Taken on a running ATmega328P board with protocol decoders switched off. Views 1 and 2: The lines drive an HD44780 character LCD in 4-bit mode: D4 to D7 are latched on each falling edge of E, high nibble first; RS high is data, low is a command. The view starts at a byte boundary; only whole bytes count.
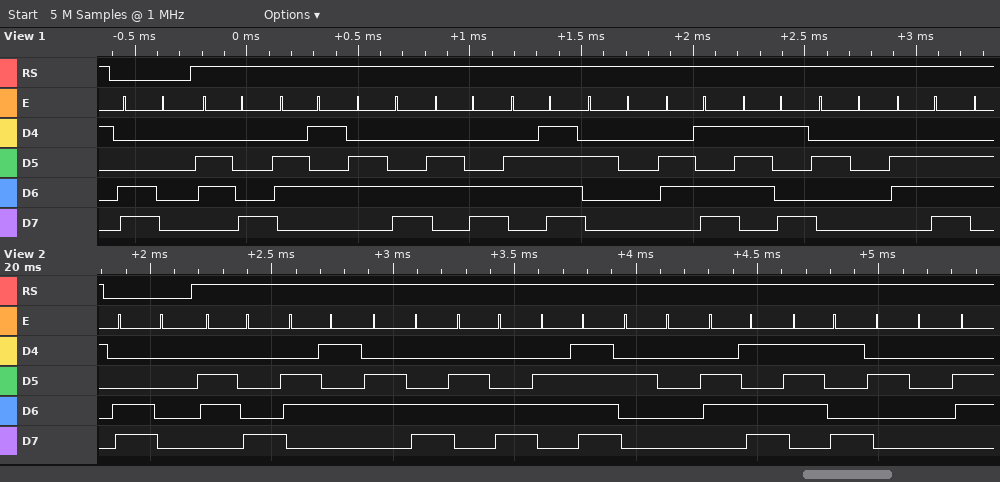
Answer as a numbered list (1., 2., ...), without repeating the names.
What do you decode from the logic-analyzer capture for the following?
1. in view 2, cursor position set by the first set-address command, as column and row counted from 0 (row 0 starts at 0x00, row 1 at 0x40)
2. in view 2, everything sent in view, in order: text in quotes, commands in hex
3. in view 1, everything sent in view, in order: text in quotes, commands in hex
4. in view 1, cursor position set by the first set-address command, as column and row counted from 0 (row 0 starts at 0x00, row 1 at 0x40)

1. column 0, row 1
2. 0xC0 "hello my "
3. 0xC0 "hello my n"
4. column 0, row 1
